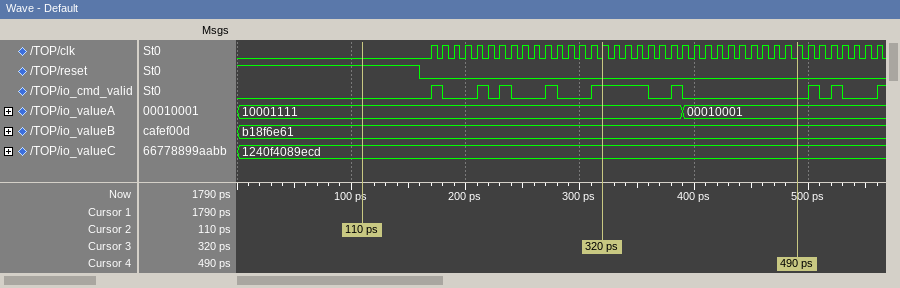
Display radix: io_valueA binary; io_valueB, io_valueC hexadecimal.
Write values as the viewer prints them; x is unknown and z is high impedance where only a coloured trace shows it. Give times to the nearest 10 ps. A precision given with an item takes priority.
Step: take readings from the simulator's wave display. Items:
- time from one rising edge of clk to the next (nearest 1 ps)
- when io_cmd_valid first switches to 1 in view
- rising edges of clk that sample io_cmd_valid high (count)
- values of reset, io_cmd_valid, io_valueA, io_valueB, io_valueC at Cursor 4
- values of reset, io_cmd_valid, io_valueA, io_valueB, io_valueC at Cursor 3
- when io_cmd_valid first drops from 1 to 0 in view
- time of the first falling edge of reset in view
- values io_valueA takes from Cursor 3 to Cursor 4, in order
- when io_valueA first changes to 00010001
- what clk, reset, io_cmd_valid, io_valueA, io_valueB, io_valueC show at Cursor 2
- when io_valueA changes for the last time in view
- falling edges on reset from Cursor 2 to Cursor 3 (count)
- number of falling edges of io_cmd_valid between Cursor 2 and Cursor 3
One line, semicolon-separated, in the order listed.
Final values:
10 ps; 170 ps; 12; reset=0, io_cmd_valid=0, io_valueA=00010001, io_valueB=b18f6e61, io_valueC=1240f4089ecd; reset=0, io_cmd_valid=1, io_valueA=10001111, io_valueB=b18f6e61, io_valueC=1240f4089ecd; 180 ps; 160 ps; 10001111, 00010001; 390 ps; clk=0, reset=1, io_cmd_valid=0, io_valueA=10001111, io_valueB=b18f6e61, io_valueC=1240f4089ecd; 390 ps; 1; 4
